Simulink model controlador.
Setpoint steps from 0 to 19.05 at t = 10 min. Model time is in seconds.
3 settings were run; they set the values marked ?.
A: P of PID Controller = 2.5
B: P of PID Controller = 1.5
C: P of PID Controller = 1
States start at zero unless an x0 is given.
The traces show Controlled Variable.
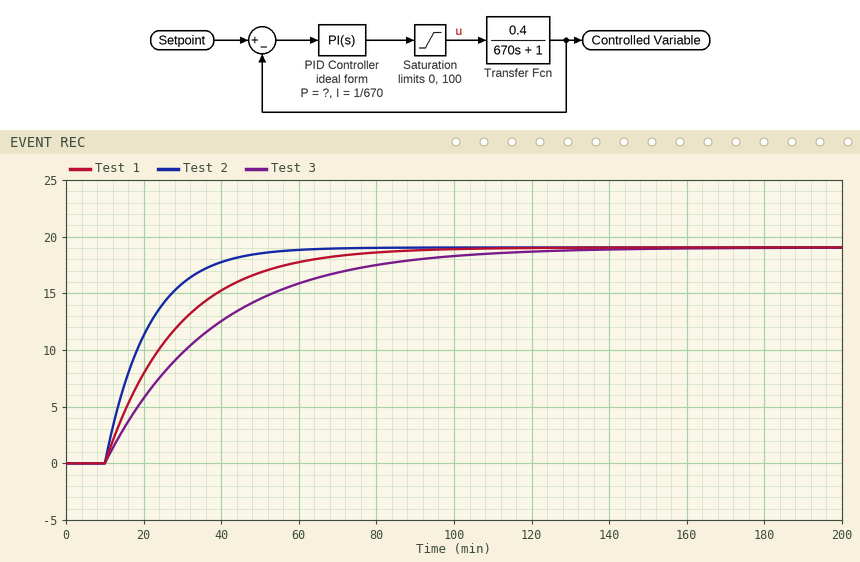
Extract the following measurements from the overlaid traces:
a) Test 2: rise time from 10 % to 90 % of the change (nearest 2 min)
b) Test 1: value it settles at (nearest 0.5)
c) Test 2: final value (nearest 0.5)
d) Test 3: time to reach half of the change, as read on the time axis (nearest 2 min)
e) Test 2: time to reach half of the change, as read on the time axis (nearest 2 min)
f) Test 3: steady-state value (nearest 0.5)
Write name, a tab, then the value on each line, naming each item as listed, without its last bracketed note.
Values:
Test 2: rise time from 10 % to 90 % of the change	24 min
Test 1: value it settles at	19.0
Test 2: final value	19.0
Test 3: time to reach half of the change, as read on the time axis	30 min
Test 2: time to reach half of the change, as read on the time axis	18 min
Test 3: steady-state value	19.0
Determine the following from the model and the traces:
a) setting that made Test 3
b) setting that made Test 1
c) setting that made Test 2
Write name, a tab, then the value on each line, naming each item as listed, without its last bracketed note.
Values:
setting that made Test 3	C
setting that made Test 1	B
setting that made Test 2	A
